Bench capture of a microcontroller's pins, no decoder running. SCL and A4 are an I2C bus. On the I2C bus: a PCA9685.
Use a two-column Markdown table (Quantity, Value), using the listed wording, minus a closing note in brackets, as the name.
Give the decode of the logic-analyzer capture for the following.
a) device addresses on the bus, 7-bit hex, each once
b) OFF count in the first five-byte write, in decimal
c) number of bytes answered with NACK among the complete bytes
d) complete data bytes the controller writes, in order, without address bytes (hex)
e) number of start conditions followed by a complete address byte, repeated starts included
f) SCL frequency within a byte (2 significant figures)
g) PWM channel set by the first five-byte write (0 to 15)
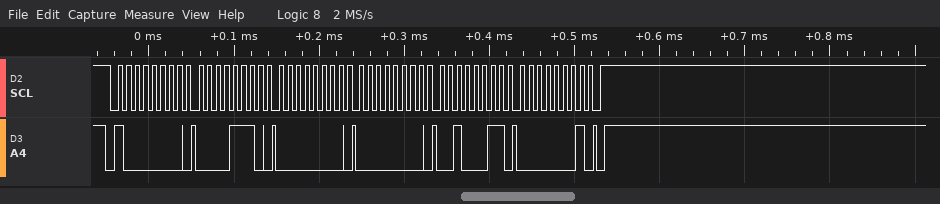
| Quantity | Value |
|---|---|
| device addresses on the bus, 7-bit hex, each once | 0x40 |
| OFF count in the first five-byte write, in decimal | 291 |
| number of bytes answered with NACK among the complete bytes | 0 |
| complete data bytes the controller writes, in order, without address bytes | 0E 00 00 23 01 |
| number of start conditions followed by a complete address byte, repeated starts included | 1 |
| SCL frequency within a byte | 100 kHz |
| PWM channel set by the first five-byte write | 2 |
